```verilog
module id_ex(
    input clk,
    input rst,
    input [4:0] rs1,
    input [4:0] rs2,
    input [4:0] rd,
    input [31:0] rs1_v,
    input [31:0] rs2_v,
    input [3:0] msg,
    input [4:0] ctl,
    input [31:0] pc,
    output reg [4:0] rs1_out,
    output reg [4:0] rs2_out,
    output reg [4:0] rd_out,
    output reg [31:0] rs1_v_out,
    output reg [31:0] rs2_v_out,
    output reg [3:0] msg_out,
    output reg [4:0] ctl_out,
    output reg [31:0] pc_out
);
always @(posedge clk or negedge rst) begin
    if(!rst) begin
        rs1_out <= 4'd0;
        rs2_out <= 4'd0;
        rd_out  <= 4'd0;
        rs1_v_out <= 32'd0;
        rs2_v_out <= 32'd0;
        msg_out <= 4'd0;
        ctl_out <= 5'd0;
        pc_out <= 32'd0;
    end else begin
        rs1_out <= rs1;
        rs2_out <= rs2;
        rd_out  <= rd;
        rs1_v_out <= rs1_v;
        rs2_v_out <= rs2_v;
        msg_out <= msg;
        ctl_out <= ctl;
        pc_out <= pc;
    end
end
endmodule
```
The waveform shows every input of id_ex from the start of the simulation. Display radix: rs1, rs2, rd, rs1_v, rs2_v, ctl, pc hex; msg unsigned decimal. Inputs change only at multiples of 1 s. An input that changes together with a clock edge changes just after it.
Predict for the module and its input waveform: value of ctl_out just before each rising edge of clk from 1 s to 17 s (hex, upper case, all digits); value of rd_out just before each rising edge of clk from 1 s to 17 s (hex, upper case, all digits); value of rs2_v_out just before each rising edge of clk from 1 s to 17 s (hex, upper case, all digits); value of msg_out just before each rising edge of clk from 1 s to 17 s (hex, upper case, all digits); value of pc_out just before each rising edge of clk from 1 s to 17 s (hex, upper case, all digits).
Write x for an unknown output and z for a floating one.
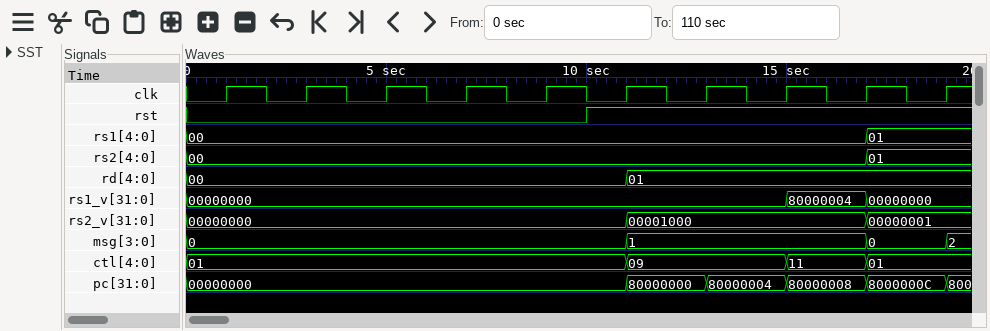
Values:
00, 00, 00, 00, 00, 00, 01, 09, 09
00, 00, 00, 00, 00, 00, 00, 01, 01
00000000, 00000000, 00000000, 00000000, 00000000, 00000000, 00000000, 00001000, 00001000
0, 0, 0, 0, 0, 0, 0, 1, 1
00000000, 00000000, 00000000, 00000000, 00000000, 00000000, 00000000, 80000000, 80000004
